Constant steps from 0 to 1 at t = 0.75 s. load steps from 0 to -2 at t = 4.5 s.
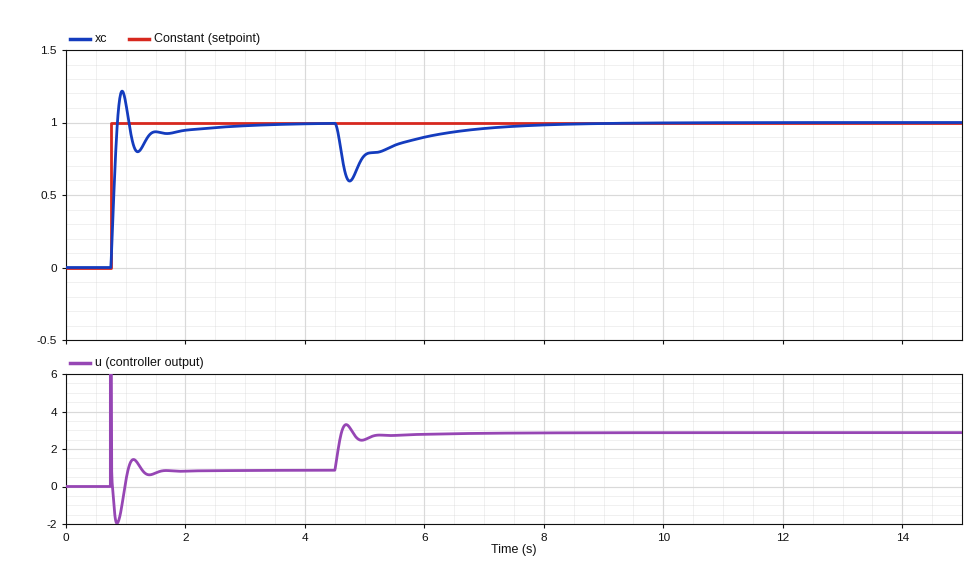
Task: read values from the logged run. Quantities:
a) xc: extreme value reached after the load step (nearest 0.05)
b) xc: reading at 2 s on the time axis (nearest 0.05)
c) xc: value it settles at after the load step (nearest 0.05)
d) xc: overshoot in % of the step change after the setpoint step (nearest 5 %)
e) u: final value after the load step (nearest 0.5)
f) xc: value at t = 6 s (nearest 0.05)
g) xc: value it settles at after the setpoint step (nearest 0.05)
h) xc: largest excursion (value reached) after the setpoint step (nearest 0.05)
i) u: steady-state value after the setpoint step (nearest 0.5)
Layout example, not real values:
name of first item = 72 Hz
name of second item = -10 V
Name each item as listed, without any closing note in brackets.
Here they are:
xc: extreme value reached after the load step = 0.60
xc: reading at 2 s on the time axis = 0.95
xc: value it settles at after the load step = 1.00
xc: overshoot in % of the step change after the setpoint step = 20 %
u: final value after the load step = 3.0
xc: value at t = 6 s = 0.90
xc: value it settles at after the setpoint step = 1.00
xc: largest excursion (value reached) after the setpoint step = 1.20
u: steady-state value after the setpoint step = 1.0
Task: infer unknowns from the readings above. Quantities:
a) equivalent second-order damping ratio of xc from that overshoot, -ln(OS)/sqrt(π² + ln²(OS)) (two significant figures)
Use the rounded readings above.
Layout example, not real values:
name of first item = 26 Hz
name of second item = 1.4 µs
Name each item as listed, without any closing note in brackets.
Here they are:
equivalent second-order damping ratio of xc from that overshoot, -ln(OS)/sqrt(π² + ln²(OS)) = 0.46
